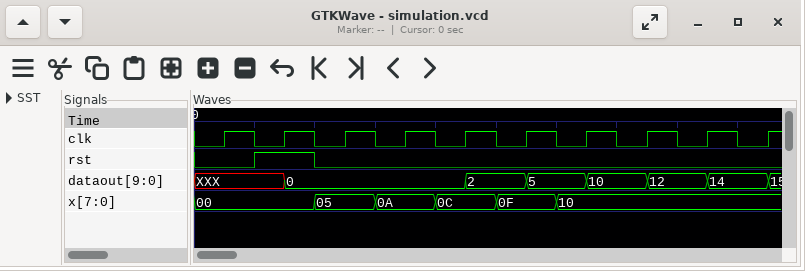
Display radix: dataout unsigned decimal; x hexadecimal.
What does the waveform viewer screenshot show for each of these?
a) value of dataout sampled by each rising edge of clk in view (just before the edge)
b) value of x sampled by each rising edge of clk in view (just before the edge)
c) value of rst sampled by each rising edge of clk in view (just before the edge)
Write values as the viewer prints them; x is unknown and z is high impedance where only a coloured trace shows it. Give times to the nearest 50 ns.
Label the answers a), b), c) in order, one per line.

a) XXX, XXX, 0, 0, 0, 2, 5, 10, 12, 14
b) 00, 00, 05, 0A, 0C, 0F, 10, 10, 10, 10
c) 0 1 0 0 0 0 0 0 0 0
